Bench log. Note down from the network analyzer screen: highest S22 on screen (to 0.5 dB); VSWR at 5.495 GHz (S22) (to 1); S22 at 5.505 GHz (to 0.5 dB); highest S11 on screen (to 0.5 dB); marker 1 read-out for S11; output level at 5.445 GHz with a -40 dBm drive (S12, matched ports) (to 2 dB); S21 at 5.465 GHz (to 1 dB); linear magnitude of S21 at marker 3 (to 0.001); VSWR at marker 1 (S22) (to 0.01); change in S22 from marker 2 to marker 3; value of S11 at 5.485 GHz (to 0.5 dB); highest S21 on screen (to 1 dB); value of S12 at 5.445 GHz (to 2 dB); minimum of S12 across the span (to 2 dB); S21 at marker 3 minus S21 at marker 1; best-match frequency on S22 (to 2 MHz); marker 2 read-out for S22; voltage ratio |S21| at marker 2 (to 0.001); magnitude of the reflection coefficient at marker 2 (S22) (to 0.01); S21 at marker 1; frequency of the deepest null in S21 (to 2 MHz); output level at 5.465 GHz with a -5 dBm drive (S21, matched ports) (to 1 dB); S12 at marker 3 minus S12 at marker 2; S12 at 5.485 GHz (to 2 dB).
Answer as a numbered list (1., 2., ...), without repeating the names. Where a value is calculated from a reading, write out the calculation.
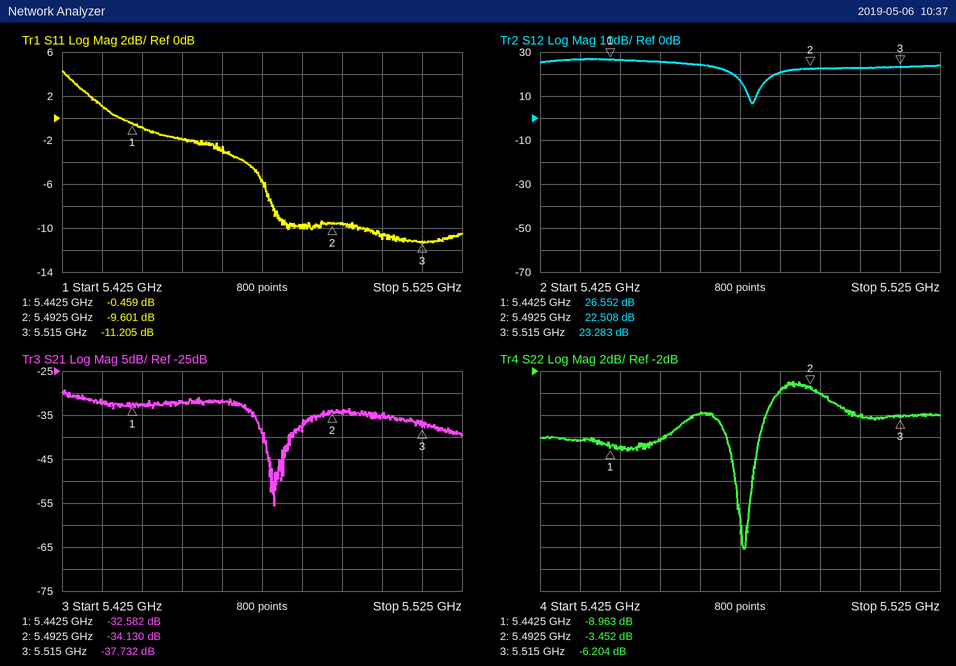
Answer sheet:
1. -3.0 dB
2. |Γ| = 10^(-4/20) = 0.6310; VSWR = (1 + 0.6310)/(1 − 0.6310) ≈ 4
3. -6.0 dB
4. 4.5 dB
5. -0.459 dB
6. -40 dBm + (26 dB) = -14 dBm
7. -32 dB
8. 10^(-37.732/20) ≈ 0.013
9. (1 + 0.3563)/(1 − 0.3563) ≈ 2.11
10. -6.204 − (-3.452) = -2.752 dB
11. -10.0 dB
12. -29 dB
13. 26 dB
14. 6 dB
15. -37.732 − (-32.582) = -5.150 dB
16. 5.476 GHz
17. -3.452 dB
18. 10^(-34.13/20) ≈ 0.020
19. 10^(-3.452/20) ≈ 0.67
20. -32.582 dB
21. 5.478 GHz
22. -5 dBm + (-32 dB) = -37 dBm
23. 23.283 − (22.508) = 0.775 dB
24. 20 dB
